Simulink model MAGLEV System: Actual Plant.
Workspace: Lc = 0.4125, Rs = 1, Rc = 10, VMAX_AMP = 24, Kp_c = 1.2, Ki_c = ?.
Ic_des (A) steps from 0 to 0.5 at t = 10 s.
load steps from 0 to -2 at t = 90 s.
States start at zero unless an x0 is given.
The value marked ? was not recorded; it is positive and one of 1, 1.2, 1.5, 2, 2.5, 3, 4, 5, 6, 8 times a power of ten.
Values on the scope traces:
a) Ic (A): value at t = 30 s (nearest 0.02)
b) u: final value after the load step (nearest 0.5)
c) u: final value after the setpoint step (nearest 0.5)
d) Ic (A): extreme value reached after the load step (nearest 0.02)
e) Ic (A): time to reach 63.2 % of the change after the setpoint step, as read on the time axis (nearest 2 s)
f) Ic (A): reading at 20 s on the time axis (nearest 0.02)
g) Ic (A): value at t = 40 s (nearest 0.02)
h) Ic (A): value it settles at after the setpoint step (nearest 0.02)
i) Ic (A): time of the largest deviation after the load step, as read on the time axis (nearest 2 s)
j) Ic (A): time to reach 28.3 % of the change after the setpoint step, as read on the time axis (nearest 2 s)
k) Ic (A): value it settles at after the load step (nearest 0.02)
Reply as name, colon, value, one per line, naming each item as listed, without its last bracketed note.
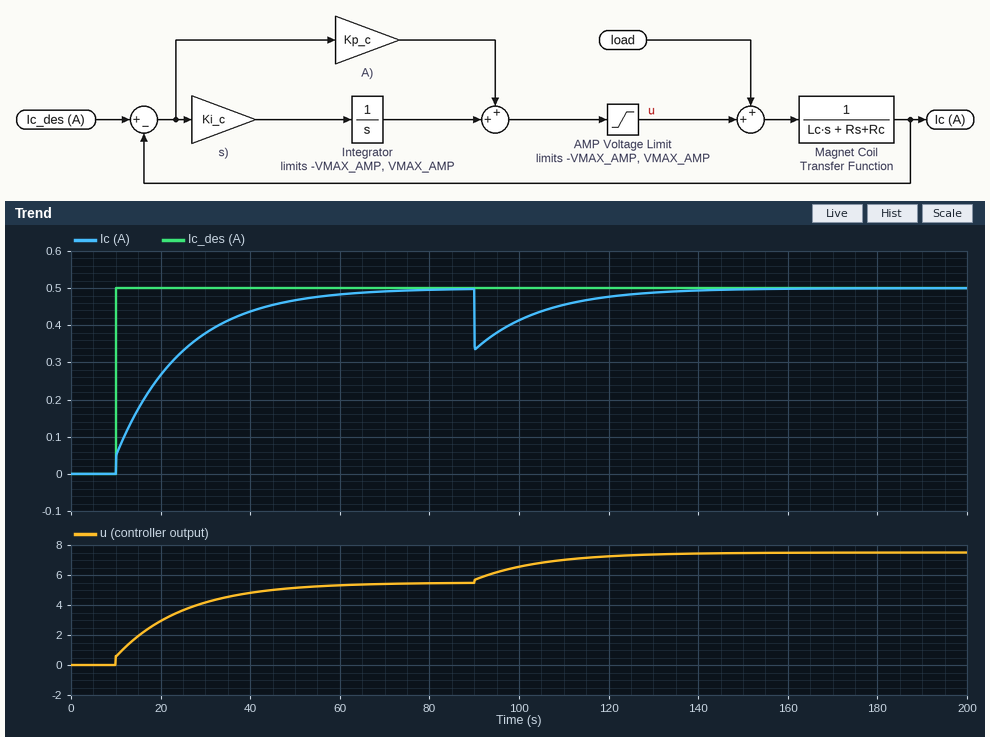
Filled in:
Ic (A): value at t = 30 s: 0.38
u: final value after the load step: 7.5
u: final value after the setpoint step: 5.5
Ic (A): extreme value reached after the load step: 0.34
Ic (A): time to reach 63.2 % of the change after the setpoint step, as read on the time axis: 24 s
Ic (A): reading at 20 s on the time axis: 0.26
Ic (A): value at t = 40 s: 0.44
Ic (A): value it settles at after the setpoint step: 0.50
Ic (A): time of the largest deviation after the load step, as read on the time axis: 90 s
Ic (A): time to reach 28.3 % of the change after the setpoint step, as read on the time axis: 14 s
Ic (A): value it settles at after the load step: 0.50
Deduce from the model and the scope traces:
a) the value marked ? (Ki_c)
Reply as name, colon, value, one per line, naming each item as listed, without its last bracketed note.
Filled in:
the value marked ?: 0.8
